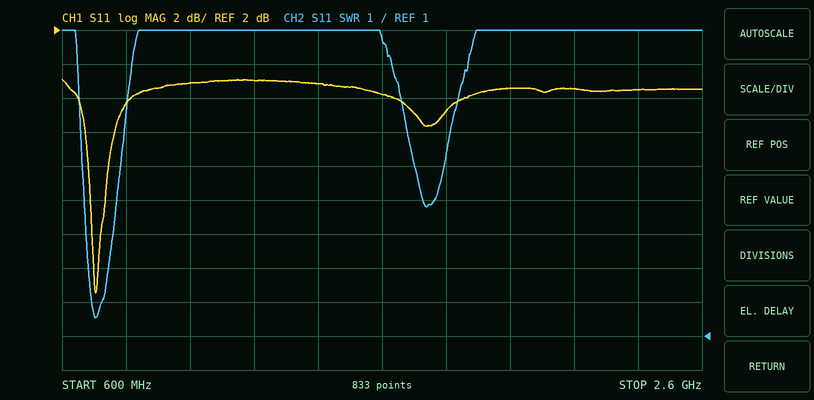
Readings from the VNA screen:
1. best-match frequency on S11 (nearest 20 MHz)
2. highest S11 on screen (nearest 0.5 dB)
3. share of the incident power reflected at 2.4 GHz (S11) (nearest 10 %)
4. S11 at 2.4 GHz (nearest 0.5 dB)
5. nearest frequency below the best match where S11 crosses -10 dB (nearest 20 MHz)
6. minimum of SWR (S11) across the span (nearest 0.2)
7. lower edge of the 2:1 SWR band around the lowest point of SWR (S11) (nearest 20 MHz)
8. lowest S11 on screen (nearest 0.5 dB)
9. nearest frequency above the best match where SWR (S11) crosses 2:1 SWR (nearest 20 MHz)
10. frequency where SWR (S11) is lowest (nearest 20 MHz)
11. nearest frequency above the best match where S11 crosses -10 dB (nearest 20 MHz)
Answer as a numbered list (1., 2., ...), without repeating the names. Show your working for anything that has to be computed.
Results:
1. 700 MHz
2. -1.0 dB
3. 10^(-1.5/10) ≈ 70.8 %, so 70 % to the nearest 10 %
4. -1.5 dB
5. 700 MHz
6. 1.6
7. 700 MHz
8. -13.5 dB
9. 720 MHz
10. 700 MHz
11. 720 MHz
